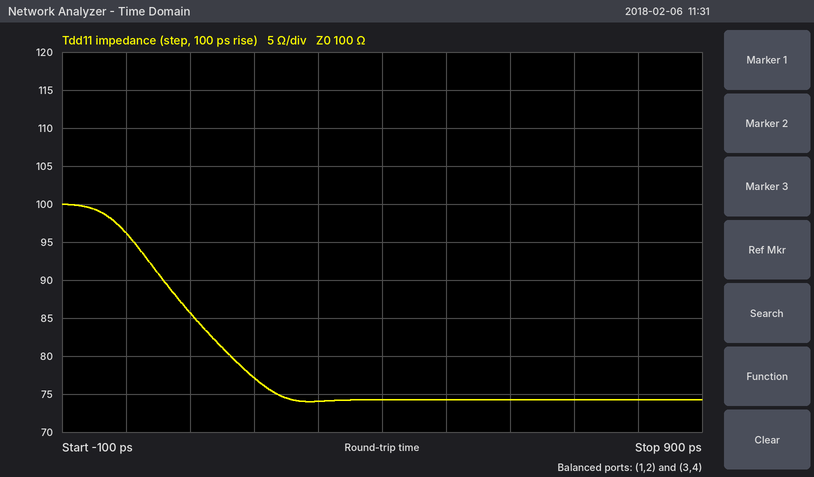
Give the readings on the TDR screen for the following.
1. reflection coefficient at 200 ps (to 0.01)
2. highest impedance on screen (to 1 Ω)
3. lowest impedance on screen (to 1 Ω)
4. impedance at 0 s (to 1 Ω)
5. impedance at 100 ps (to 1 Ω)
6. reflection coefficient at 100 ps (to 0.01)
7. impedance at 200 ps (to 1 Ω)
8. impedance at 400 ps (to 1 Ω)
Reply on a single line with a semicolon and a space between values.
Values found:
-0.13; 100 Ω; 74 Ω; 96 Ω; 86 Ω; -0.08; 77 Ω; 74 Ω
